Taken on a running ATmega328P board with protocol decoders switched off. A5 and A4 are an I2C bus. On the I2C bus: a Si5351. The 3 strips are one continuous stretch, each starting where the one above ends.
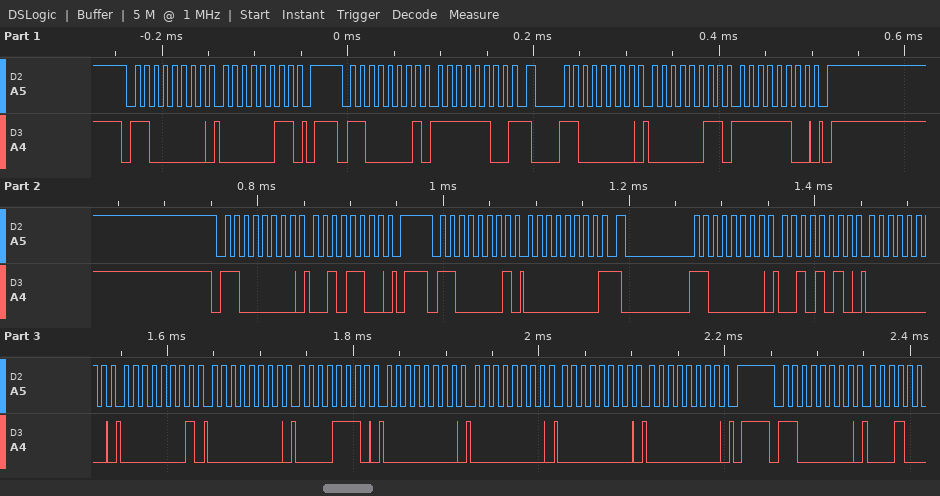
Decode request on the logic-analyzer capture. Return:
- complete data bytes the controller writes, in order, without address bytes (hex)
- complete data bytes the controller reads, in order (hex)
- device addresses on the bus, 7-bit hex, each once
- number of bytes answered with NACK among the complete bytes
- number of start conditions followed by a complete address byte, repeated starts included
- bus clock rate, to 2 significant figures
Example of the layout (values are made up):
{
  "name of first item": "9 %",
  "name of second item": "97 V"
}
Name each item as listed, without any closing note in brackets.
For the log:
{
  "complete data bytes the controller writes, in order, without address bytes": "03 03 FC 2C 2A 00 01 00 0E 00 00 00 00",
  "complete data bytes the controller reads, in order": "FC 00",
  "device addresses on the bus, 7-bit hex, each once": "0x60",
  "number of bytes answered with NACK among the complete bytes": "2",
  "number of start conditions followed by a complete address byte, repeated starts included": "7",
  "bus clock rate, to 2 significant figures": "100 kHz"
}
